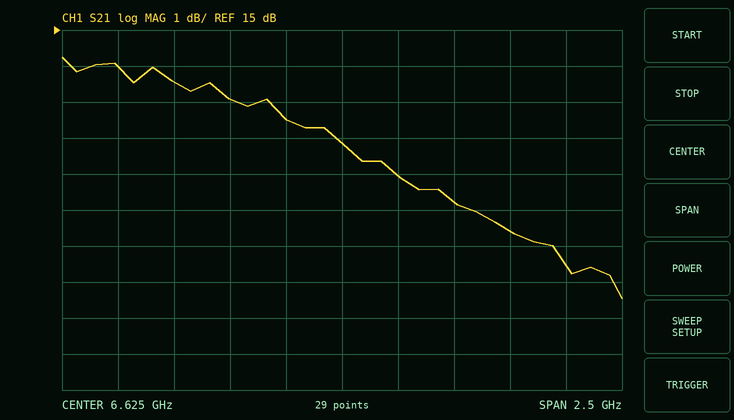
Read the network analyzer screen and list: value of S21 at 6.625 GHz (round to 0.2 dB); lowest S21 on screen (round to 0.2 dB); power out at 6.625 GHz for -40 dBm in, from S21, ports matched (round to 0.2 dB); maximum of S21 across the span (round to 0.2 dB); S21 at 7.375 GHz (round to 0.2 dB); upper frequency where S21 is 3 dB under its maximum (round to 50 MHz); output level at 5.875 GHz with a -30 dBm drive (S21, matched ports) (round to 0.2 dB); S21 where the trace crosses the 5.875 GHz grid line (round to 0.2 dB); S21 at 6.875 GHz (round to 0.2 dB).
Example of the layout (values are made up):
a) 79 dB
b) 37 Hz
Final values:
a) 11.8 dB
b) 7.6 dB
c) -28.2 dBm
d) 14.2 dB
e) 9.4 dB
f) 6.80 GHz
g) -16.4 dBm
h) 13.6 dB
i) 11.0 dB
